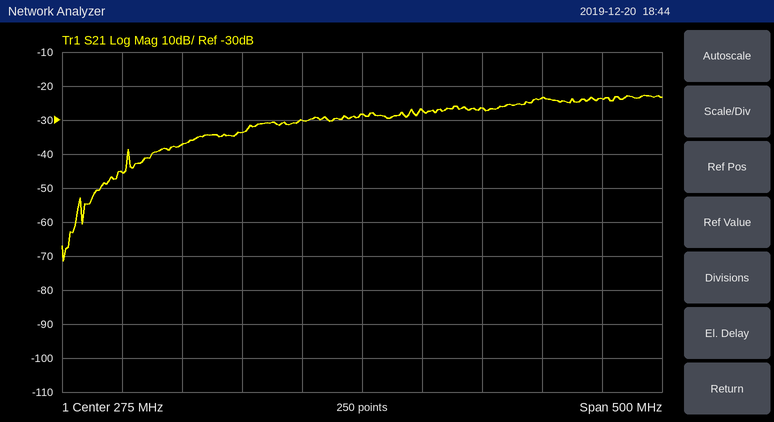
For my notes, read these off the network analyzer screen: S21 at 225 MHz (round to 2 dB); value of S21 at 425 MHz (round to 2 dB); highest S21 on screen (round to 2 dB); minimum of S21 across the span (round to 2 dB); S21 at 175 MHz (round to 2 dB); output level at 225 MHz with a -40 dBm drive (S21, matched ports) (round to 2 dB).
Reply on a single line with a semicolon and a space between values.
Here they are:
-30 dB; -24 dB; -22 dB; -72 dB; -34 dB; -70 dBm
